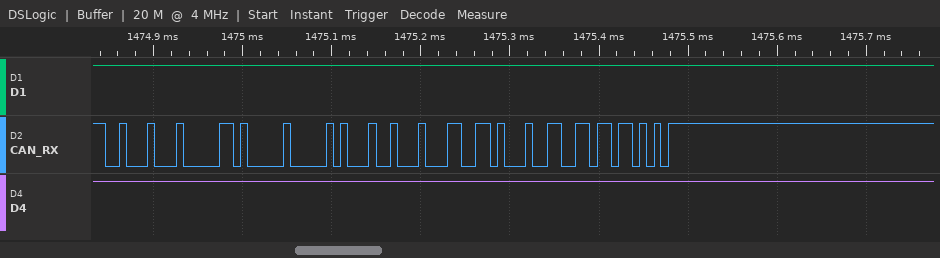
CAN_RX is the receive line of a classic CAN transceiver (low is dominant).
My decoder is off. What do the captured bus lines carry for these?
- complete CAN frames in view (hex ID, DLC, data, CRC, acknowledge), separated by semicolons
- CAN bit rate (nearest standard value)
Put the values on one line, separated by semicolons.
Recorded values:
ID 222, DLC 5, data 00 11 22 33 44, CRC 66DA, ACK; 125 kbit/s
